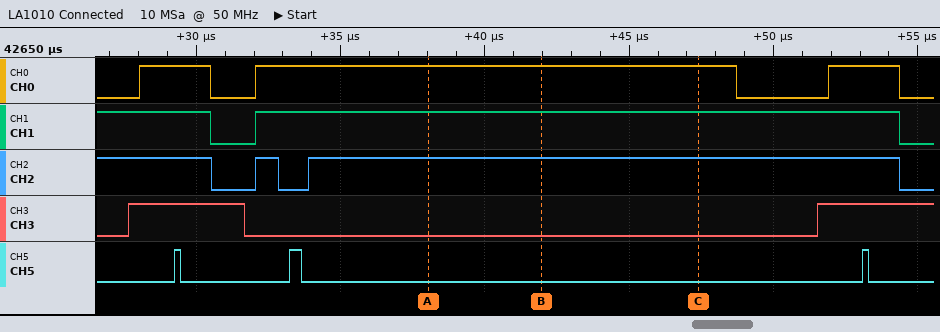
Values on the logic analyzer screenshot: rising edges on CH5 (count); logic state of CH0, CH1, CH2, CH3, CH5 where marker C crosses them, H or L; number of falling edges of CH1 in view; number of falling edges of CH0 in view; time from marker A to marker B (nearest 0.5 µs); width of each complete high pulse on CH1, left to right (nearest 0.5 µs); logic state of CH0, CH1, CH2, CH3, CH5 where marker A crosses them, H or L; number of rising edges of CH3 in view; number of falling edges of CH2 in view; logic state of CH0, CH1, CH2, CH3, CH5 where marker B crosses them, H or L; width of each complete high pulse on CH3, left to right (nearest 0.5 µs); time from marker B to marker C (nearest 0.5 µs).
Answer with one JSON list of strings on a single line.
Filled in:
["3", "CH0=H, CH1=H, CH2=H, CH3=L, CH5=L", "2", "3", "4 µs", "22.5 µs", "CH0=H, CH1=H, CH2=H, CH3=L, CH5=L", "2", "3", "CH0=H, CH1=H, CH2=H, CH3=L, CH5=L", "4 µs", "5.5 µs"]
